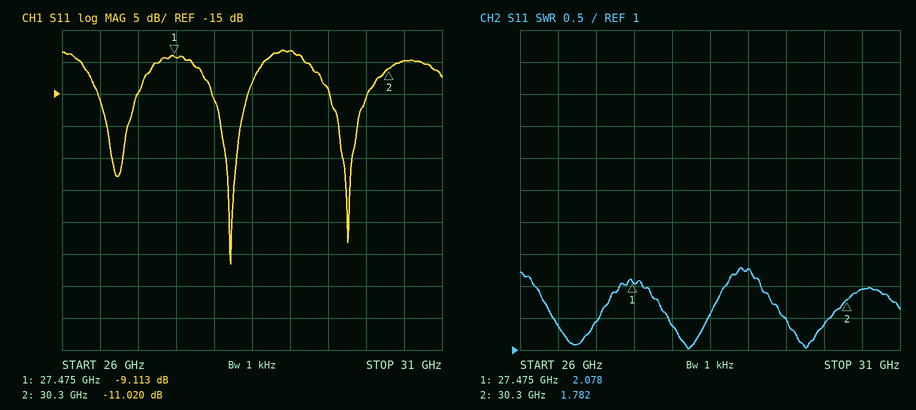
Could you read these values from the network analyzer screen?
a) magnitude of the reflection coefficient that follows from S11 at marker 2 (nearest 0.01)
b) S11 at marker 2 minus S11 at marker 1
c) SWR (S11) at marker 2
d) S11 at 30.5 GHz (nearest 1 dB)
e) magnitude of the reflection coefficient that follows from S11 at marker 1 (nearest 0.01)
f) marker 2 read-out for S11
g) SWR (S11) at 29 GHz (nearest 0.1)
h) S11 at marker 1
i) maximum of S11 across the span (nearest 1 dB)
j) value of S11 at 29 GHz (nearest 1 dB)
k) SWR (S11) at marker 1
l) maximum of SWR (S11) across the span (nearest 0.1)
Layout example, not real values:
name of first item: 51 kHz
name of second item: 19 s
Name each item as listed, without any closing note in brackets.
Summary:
magnitude of the reflection coefficient that follows from S11 at marker 2: 0.28
S11 at marker 2 minus S11 at marker 1: -1.907 dB
SWR (S11) at marker 2: 1.782
S11 at 30.5 GHz: -10 dB
magnitude of the reflection coefficient that follows from S11 at marker 1: 0.35
marker 2 read-out for S11: -11.020 dB
SWR (S11) at 29 GHz: 2.3
S11 at marker 1: -9.113 dB
maximum of S11 across the span: -8 dB
value of S11 at 29 GHz: -8 dB
SWR (S11) at marker 1: 2.078
maximum of SWR (S11) across the span: 2.3
